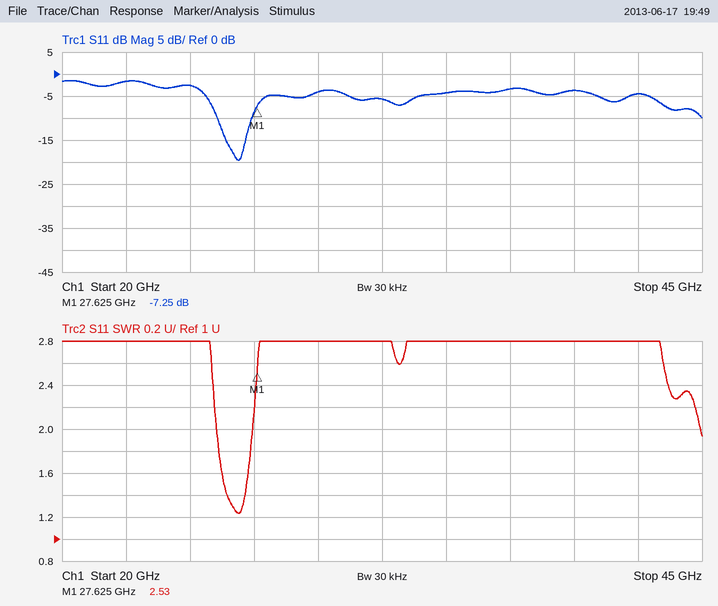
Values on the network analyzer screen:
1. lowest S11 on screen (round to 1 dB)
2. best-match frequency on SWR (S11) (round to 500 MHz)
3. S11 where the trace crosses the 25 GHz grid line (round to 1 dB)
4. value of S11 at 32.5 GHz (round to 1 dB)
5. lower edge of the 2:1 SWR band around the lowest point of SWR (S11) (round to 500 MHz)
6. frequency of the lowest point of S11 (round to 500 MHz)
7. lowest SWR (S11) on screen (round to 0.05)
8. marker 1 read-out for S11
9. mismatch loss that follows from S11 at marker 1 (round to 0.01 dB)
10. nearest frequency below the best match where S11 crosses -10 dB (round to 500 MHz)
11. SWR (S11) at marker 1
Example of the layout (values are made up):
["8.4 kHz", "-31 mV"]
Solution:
["-20 dB", "27.0 GHz", "-3 dB", "-6 dB", "26.0 GHz", "27.0 GHz", "1.25", "-7.25 dB", "0.91 dB", "26.0 GHz", "2.53"]
